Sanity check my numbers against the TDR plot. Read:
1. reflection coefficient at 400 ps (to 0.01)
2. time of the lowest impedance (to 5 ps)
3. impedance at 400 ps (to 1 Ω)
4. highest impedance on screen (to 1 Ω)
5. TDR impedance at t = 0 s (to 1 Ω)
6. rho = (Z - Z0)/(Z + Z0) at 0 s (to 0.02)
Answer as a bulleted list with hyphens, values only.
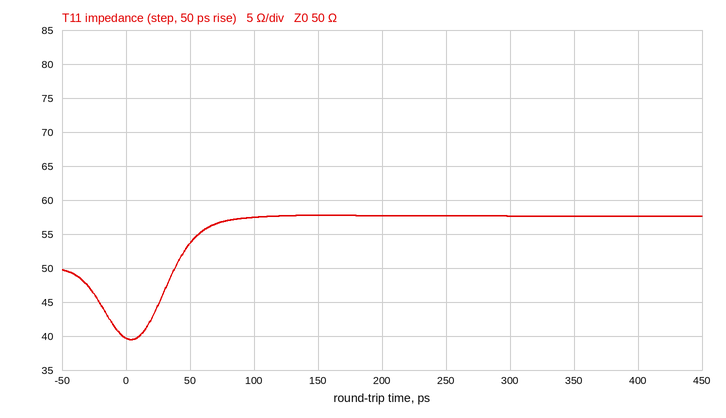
- +0.07
- 5 ps
- 58 Ω
- 58 Ω
- 40 Ω
- -0.12
